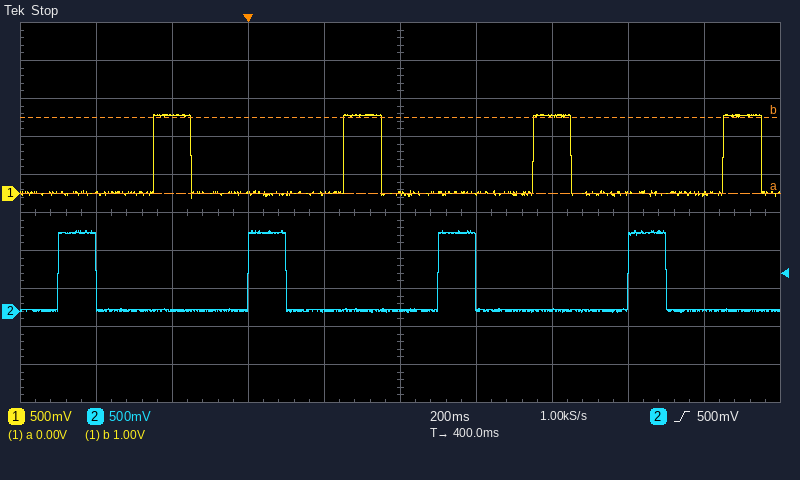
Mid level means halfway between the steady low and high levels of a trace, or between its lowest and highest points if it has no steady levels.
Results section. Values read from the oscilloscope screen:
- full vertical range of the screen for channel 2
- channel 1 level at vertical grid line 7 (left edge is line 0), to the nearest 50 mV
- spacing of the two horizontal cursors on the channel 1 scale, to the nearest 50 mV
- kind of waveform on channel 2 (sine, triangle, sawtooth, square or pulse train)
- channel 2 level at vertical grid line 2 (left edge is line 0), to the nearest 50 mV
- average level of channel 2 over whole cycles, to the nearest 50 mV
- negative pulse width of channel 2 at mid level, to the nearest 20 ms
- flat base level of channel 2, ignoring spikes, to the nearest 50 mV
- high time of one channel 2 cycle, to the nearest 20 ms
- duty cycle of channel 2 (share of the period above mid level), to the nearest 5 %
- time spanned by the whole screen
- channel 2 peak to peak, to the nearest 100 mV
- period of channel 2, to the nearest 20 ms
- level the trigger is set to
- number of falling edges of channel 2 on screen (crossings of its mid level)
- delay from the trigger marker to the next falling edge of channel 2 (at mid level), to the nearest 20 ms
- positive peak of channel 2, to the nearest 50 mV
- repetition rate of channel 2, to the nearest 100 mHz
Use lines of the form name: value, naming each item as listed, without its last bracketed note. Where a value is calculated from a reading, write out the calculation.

full vertical range of the screen for channel 2: 5 V
channel 1 level at vertical grid line 7 (left edge is line 0), to the nearest 50 mV: 1.00 V
spacing of the two horizontal cursors on the channel 1 scale, to the nearest 50 mV: 1.00 V
kind of waveform on channel 2: pulse train
channel 2 level at vertical grid line 2 (left edge is line 0), to the nearest 50 mV: 0 mV
average level of channel 2 over whole cycles, to the nearest 50 mV: 0 mV + 0.2 × (1.05 V − (0 mV)) ≈ 210 mV, so 200 mV to the nearest 50 mV
negative pulse width of channel 2 at mid level, to the nearest 20 ms: 400 ms
flat base level of channel 2, ignoring spikes, to the nearest 50 mV: 0 mV
high time of one channel 2 cycle, to the nearest 20 ms: 100 ms
duty cycle of channel 2 (share of the period above mid level), to the nearest 5 %: 100 ms / 500 ms ≈ 20 %
time spanned by the whole screen: 2 s
channel 2 peak to peak, to the nearest 100 mV: 1.10 V
period of channel 2, to the nearest 20 ms: 500 ms
level the trigger is set to: 500 mV
number of falling edges of channel 2 on screen: 4
delay from the trigger marker to the next falling edge of channel 2 (at mid level), to the nearest 20 ms: 100 ms
positive peak of channel 2, to the nearest 50 mV: 1.05 V
repetition rate of channel 2, to the nearest 100 mHz: 1 / 500 ms ≈ 2.0 Hz
